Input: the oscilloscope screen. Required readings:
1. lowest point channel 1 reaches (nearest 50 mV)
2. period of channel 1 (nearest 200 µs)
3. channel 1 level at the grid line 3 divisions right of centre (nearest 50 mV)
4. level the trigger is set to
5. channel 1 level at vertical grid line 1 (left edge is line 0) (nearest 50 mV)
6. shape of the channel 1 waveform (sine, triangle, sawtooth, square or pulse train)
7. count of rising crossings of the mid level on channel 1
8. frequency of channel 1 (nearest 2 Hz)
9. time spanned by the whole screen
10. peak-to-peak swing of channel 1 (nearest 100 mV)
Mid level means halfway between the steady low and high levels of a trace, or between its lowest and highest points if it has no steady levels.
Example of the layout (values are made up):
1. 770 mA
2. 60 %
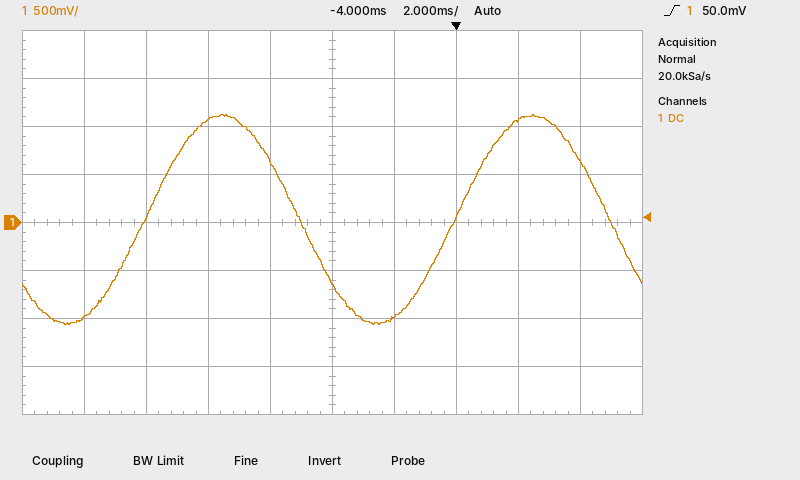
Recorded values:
1. -1.05 V
2. 10.0 ms
3. 1.05 V
4. 50.0 mV
5. -1.00 V
6. sine
7. 2
8. 100 Hz
9. 20 ms
10. 2.20 V
